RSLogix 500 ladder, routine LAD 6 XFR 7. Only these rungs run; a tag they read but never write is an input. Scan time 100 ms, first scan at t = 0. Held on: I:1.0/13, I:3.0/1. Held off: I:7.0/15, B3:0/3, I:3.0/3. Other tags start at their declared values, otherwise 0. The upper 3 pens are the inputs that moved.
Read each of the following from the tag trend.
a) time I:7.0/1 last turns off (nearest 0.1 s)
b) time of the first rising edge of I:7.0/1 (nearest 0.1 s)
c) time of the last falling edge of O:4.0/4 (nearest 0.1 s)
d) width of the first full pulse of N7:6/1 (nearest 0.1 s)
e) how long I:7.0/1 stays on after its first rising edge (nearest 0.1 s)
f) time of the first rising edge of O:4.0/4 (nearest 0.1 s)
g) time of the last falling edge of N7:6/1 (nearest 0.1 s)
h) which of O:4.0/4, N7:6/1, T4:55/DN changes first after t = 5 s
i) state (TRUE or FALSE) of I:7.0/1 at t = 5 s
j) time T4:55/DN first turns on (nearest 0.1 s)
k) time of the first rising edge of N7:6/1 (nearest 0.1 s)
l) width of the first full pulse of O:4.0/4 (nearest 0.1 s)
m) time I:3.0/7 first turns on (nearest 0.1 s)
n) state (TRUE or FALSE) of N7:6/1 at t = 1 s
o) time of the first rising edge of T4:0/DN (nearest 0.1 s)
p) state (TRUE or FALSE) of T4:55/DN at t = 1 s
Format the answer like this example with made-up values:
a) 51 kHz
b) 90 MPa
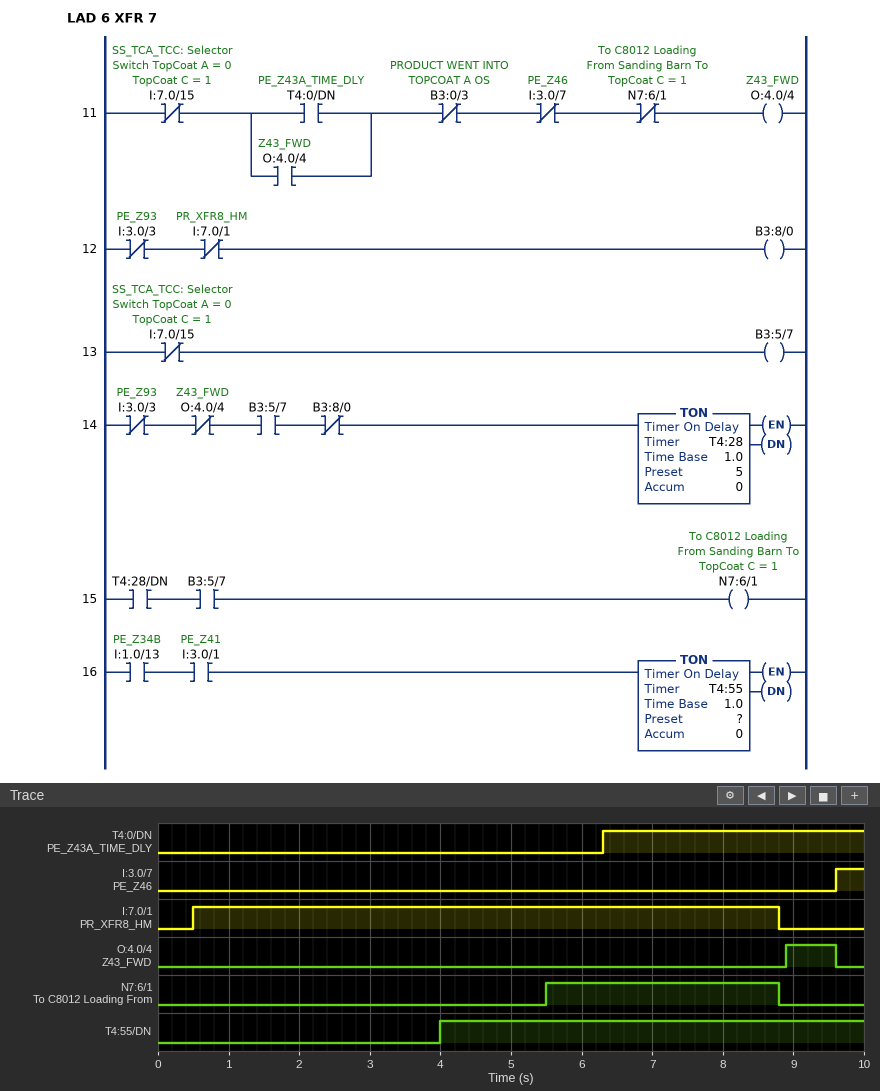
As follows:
a) 8.8 s
b) 0.5 s
c) 9.6 s
d) 3.3 s
e) 8.3 s
f) 8.9 s
g) 8.8 s
h) N7:6/1
i) TRUE
j) 4.0 s
k) 5.5 s
l) 0.7 s
m) 9.6 s
n) FALSE
o) 6.3 s
p) FALSE
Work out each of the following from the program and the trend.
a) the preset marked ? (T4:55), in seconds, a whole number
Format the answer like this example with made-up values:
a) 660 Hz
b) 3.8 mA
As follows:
a) 4 s
